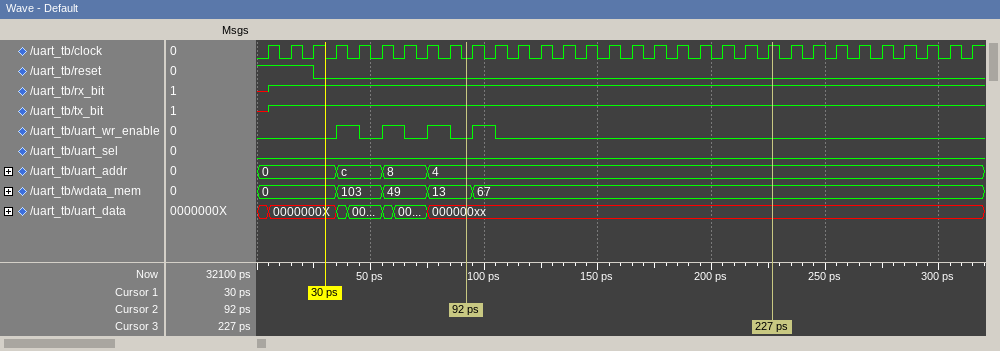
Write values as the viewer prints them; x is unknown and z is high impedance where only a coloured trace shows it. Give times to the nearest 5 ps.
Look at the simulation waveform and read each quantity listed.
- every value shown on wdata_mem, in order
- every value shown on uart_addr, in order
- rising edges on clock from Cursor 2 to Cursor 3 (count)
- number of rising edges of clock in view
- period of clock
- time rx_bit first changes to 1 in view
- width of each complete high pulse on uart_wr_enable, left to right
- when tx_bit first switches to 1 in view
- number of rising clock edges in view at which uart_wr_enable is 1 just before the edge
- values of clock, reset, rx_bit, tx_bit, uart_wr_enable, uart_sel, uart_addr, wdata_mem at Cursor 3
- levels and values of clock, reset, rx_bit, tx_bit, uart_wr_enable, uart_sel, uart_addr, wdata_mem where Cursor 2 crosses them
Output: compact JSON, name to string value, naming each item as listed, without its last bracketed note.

{"every value shown on wdata_mem, in order": "0, 103, 49, 13, 67", "every value shown on uart_addr, in order": "0, c, 8, 4", "rising edges on clock from Cursor 2 to Cursor 3": "14", "number of rising edges of clock in view": "32", "period of clock": "10 ps", "time rx_bit first changes to 1 in view": "5 ps", "width of each complete high pulse on uart_wr_enable, left to right": "10 ps, 10 ps, 10 ps, 10 ps", "when tx_bit first switches to 1 in view": "5 ps", "number of rising clock edges in view at which uart_wr_enable is 1 just before the edge": "4", "values of clock, reset, rx_bit, tx_bit, uart_wr_enable, uart_sel, uart_addr, wdata_mem at Cursor 3": "clock=1, reset=0, rx_bit=1, tx_bit=1, uart_wr_enable=0, uart_sel=0, uart_addr=4, wdata_mem=67", "levels and values of clock, reset, rx_bit, tx_bit, uart_wr_enable, uart_sel, uart_addr, wdata_mem where Cursor 2 crosses them": "clock=0, reset=0, rx_bit=1, tx_bit=1, uart_wr_enable=0, uart_sel=0, uart_addr=4, wdata_mem=13"}
